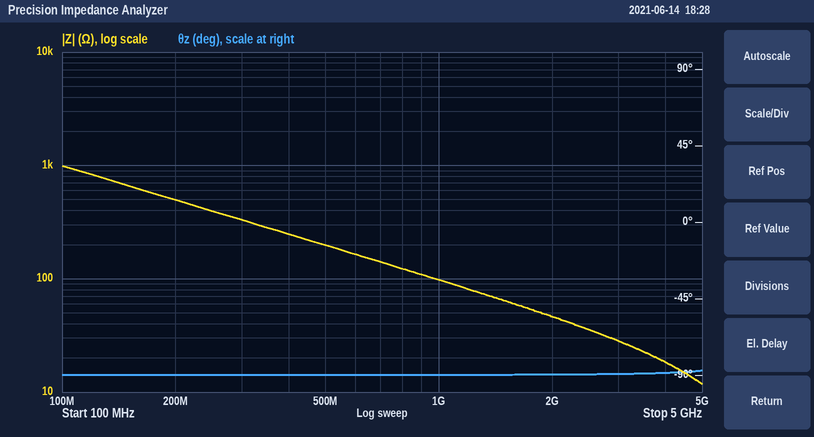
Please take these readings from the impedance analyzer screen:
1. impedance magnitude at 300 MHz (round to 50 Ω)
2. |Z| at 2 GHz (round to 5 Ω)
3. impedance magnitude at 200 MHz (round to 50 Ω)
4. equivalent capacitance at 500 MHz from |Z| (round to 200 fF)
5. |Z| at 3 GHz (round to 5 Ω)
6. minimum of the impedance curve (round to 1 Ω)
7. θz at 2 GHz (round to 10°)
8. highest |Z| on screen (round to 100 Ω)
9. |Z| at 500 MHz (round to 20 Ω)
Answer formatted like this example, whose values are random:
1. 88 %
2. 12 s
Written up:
1. 350 Ω
2. 45 Ω
3. 500 Ω
4. 1.6 pF
5. 30 Ω
6. 12 Ω
7. -90°
8. 1.0 kΩ
9. 200 Ω
